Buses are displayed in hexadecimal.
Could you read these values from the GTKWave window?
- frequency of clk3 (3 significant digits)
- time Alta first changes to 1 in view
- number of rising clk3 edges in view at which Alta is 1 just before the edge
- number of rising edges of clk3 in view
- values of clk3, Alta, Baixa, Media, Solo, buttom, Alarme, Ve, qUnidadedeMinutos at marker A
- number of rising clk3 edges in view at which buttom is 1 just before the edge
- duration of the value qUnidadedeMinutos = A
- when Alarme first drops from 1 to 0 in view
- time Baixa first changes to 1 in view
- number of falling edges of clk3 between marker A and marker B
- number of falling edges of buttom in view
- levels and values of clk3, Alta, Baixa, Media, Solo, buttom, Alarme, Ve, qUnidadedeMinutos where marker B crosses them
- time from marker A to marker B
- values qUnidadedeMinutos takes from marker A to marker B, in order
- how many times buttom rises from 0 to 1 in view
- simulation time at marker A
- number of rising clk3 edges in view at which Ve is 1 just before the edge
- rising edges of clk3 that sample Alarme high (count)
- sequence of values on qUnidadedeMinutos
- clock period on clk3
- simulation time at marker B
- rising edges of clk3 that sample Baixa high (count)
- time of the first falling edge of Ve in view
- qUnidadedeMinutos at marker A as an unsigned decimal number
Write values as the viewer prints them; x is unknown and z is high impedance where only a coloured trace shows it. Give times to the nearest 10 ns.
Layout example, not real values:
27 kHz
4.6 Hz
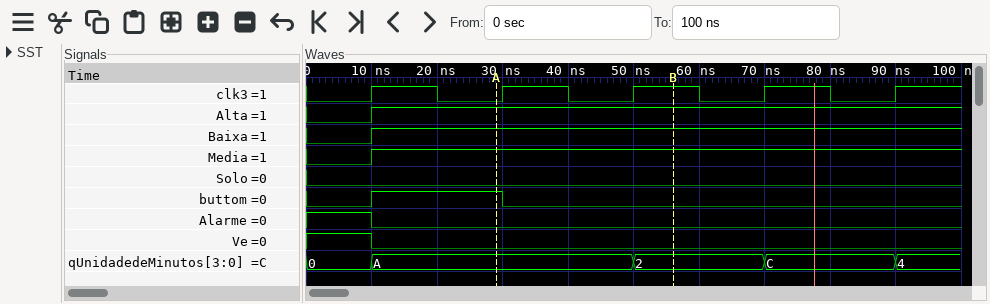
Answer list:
50.0 MHz
10 ns
4
5
clk3=0, Alta=1, Baixa=1, Media=1, Solo=0, buttom=1, Alarme=0, Ve=0, qUnidadedeMinutos=A
1
40 ns
10 ns
10 ns
1
1
clk3=1, Alta=1, Baixa=1, Media=1, Solo=0, buttom=0, Alarme=0, Ve=0, qUnidadedeMinutos=2
30 ns
A, 2
1
30 ns
1
1
0, A, 2, C, 4
20 ns
60 ns
4
10 ns
10
